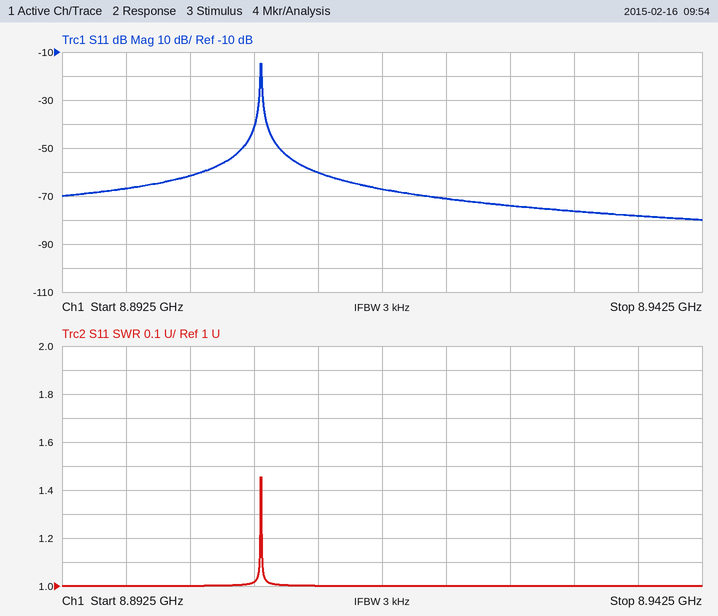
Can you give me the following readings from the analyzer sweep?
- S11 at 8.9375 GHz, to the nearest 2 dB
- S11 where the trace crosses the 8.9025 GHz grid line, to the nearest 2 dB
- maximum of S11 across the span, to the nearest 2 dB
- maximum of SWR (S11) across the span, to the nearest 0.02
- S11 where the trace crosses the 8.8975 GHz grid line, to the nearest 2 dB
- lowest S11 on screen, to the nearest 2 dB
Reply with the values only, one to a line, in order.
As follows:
-78 dB
-62 dB
-14 dB
1.46
-66 dB
-80 dB
